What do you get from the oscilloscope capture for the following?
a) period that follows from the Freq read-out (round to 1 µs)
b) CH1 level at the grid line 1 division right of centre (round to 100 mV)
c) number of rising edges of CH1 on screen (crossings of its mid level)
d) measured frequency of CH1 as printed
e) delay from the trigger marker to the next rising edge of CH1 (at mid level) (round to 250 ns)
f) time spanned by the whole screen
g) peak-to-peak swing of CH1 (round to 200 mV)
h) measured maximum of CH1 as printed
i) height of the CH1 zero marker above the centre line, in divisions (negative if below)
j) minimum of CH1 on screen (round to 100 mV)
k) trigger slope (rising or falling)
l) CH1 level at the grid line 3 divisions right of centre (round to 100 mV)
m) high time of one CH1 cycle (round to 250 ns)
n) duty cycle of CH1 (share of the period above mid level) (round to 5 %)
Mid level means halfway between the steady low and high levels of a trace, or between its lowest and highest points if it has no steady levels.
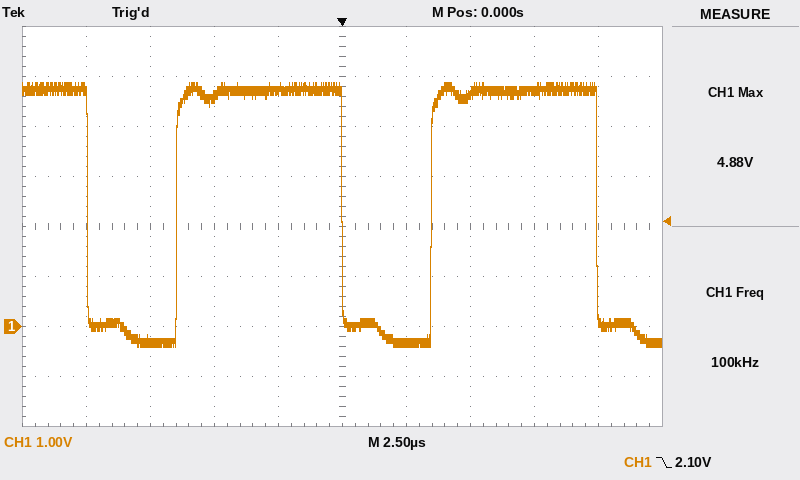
10 µs
-300 mV
2
100 kHz
3.50 µs
25 µs
5.2 V
4.88 V
-2.0 div
-400 mV
falling
4.7 V
6.50 µs
65 %
